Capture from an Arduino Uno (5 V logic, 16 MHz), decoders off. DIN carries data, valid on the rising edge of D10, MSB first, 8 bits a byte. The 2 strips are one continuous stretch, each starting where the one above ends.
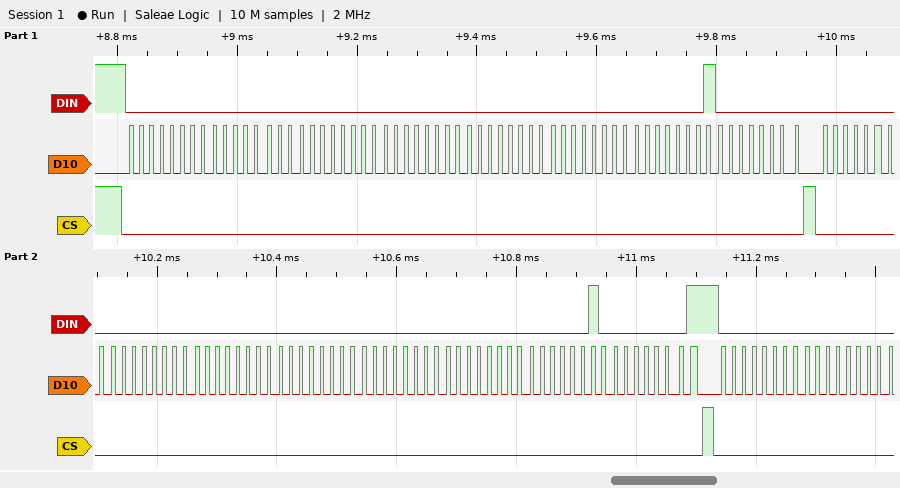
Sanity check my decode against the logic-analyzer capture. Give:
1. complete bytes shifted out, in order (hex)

00 00 00 00 00 00 01 00 00 00 00 00 00 00 02 01 00 00
